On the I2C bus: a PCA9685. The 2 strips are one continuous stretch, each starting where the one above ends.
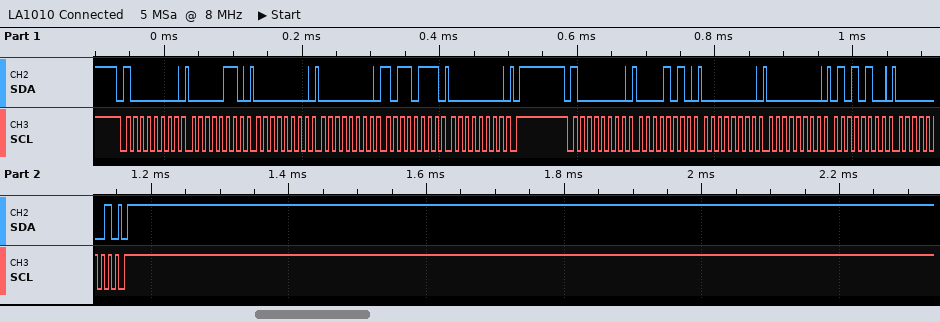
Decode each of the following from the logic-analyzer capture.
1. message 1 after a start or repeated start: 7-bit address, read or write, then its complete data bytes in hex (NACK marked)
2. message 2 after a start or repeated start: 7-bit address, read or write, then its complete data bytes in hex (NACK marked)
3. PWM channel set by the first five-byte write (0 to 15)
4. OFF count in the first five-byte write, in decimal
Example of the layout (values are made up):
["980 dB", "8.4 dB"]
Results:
["0x40 write: 06 00 00 B7 00", "0x40 write: 0A 00 00 54 01", "0", "183"]
